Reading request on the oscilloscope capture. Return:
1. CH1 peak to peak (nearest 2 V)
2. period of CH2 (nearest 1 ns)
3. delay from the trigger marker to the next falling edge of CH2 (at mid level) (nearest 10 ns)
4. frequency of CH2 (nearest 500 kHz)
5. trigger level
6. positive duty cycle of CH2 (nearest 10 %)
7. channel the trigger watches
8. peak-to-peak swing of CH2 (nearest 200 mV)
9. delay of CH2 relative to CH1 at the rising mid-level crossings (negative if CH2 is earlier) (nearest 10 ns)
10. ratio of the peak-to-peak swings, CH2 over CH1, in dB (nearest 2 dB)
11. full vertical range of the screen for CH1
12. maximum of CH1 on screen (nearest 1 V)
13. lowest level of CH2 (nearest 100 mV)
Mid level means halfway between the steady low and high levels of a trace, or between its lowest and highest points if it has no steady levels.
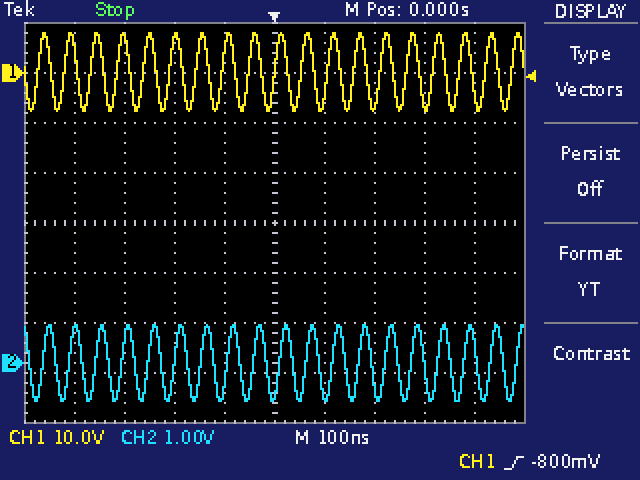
16 V
53 ns
40 ns
19.0 MHz
-800 mV
50 %
CH1
1.6 V
+10 ns
-20 dB
80 V
8 V
-800 mV
